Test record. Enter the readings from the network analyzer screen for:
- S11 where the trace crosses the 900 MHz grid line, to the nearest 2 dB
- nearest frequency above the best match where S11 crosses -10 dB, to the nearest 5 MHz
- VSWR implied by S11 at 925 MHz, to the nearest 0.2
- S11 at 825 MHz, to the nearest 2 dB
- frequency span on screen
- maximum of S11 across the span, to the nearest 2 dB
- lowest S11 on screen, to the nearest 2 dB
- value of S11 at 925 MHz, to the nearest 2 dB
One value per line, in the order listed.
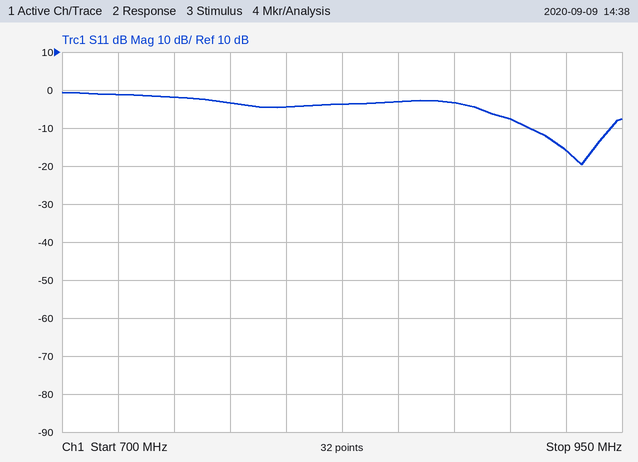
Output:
-8 dB
945 MHz
1.4
-4 dB
250 MHz
0 dB
-20 dB
-16 dB
